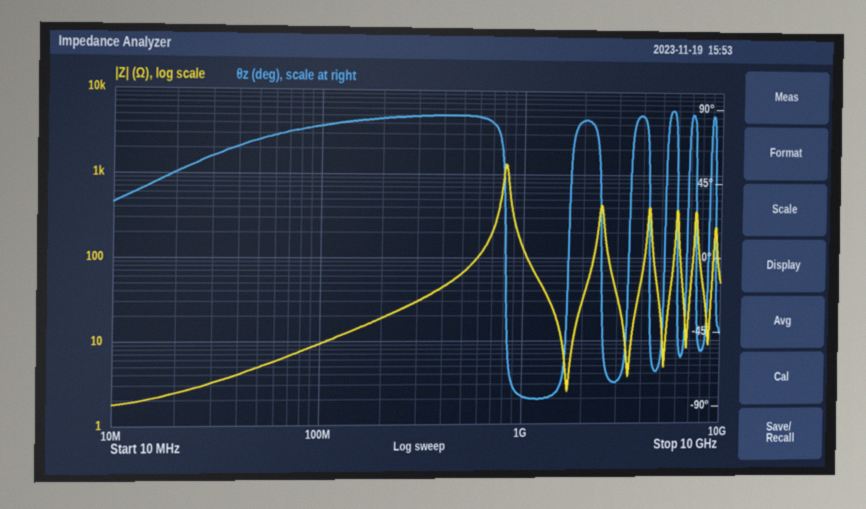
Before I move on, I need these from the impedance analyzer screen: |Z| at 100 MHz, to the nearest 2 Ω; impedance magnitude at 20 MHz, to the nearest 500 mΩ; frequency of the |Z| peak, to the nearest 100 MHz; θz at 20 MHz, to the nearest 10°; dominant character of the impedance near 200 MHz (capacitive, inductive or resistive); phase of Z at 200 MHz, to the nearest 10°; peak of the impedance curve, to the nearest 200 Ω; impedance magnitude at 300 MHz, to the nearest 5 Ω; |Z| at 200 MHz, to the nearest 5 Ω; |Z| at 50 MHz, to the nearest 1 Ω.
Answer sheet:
10 Ω
2.5 Ω
800 MHz
50°
inductive
80°
1.4 kΩ
30 Ω
20 Ω
5 Ω
